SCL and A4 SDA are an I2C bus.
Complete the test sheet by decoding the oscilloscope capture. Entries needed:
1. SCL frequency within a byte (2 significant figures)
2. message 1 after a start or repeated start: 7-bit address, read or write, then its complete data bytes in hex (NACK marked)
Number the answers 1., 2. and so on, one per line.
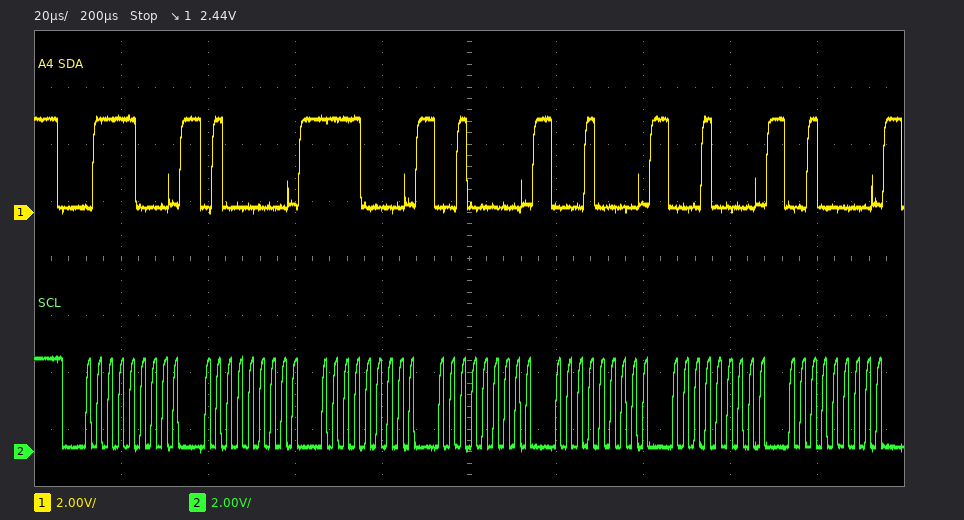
1. 400 kHz
2. 0x3C write: 40 F0 20 10 10 20
